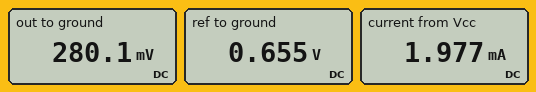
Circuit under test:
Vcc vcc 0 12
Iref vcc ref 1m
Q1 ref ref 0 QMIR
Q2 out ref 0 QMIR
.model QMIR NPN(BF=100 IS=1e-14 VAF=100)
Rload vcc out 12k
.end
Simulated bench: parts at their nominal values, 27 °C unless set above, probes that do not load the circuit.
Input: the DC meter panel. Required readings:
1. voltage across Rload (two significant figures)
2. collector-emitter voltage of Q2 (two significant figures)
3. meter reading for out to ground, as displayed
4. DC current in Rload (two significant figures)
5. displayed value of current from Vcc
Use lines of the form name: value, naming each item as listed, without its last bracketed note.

voltage across Rload: 12 V
collector-emitter voltage of Q2: 280 mV
meter reading for out to ground, as displayed: 280.1 mV
DC current in Rload: 980 µA
displayed value of current from Vcc: 1.977 mA
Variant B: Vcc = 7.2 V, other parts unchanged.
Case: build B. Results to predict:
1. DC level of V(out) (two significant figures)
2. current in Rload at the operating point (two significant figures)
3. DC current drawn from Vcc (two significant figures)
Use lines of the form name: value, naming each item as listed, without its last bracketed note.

DC level of V(out): 49 mV
current in Rload at the operating point: 600 µA
DC current drawn from Vcc: 1.6 mA
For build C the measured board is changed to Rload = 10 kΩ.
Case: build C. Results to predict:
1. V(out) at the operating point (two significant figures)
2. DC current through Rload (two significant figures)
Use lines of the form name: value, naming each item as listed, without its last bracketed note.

V(out) at the operating point: 2.1 V
DC current through Rload: 990 µA
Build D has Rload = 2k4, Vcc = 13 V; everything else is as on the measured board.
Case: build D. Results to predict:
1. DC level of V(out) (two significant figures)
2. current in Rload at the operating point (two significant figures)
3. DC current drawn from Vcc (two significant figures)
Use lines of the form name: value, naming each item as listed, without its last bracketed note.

DC level of V(out): 10 V
current in Rload at the operating point: 1.1 mA
DC current drawn from Vcc: 2.1 mA
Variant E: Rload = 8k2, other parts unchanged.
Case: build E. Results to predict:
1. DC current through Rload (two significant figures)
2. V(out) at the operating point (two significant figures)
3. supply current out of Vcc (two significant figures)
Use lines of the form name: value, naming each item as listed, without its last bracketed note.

DC current through Rload: 1.0 mA
V(out) at the operating point: 3.7 V
supply current out of Vcc: 2.0 mA
